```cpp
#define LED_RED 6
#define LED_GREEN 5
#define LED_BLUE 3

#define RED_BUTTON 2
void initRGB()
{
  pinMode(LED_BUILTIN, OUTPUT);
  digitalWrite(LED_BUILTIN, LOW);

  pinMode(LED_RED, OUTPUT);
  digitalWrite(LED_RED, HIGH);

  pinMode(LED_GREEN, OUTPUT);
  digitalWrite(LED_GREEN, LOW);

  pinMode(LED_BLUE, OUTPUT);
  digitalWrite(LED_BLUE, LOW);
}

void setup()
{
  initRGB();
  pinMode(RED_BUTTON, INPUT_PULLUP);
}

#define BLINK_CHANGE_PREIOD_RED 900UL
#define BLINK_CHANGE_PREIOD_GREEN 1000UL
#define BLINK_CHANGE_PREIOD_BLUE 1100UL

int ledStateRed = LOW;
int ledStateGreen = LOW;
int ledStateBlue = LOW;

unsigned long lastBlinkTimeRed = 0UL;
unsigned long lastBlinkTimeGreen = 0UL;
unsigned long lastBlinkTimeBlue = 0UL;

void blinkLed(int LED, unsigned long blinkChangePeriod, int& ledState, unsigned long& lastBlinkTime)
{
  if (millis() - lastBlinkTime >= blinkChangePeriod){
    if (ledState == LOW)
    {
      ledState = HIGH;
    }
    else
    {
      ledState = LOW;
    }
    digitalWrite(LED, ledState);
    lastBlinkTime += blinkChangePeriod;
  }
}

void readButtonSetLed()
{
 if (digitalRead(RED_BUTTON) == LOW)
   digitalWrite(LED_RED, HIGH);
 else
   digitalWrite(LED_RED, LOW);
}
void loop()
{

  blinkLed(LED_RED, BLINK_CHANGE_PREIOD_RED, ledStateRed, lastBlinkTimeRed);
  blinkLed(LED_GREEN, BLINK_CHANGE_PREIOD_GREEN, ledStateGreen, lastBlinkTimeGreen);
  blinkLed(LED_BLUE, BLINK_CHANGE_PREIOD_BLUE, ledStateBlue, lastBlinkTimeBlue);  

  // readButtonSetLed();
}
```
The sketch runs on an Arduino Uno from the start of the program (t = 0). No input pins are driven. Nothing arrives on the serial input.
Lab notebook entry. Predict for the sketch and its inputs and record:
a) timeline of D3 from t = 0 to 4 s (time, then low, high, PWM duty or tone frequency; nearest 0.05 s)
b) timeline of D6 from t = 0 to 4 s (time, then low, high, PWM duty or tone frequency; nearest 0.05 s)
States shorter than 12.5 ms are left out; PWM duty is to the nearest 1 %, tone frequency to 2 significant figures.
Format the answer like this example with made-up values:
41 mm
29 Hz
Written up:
0 s low; 1.1 s high; 2.2 s low; 3.3 s high
0 s high; 1.8 s low; 2.7 s high; 3.6 s low
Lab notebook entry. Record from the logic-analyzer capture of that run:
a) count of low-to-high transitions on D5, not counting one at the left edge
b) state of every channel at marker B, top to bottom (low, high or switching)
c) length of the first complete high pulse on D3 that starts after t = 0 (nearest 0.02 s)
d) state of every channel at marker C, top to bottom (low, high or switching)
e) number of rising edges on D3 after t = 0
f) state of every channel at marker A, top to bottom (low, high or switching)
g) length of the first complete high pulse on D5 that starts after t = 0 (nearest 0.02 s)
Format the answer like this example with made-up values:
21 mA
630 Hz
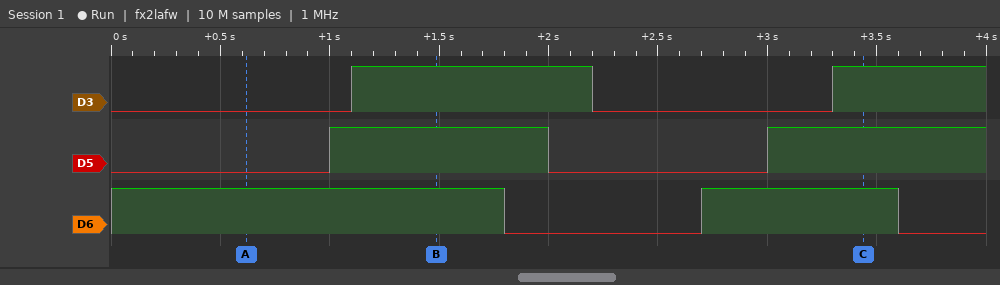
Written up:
2
D3 high, D5 high, D6 high
1.10 s
D3 high, D5 high, D6 high
2
D3 low, D5 low, D6 high
1.00 s
